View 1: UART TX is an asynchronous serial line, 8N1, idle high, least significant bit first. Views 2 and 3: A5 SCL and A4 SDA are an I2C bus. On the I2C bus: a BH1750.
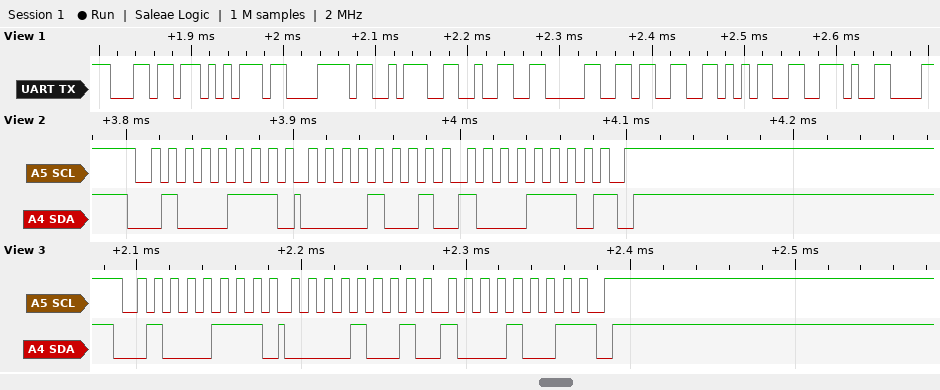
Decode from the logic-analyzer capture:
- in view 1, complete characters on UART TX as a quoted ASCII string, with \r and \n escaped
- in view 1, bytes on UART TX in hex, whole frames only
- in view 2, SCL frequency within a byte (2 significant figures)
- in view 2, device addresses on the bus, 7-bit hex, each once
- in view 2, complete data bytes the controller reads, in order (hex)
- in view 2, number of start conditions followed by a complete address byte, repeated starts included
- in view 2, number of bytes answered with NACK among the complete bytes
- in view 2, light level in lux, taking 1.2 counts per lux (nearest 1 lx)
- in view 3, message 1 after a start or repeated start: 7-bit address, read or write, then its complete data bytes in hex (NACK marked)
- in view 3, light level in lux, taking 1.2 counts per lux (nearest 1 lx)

"lux:2035."
6C 75 78 3A 32 30 33 35 2E
100 kHz
0x23
09 8E
1
1
2038 lx
0x23 read: 09 89 NACK
2034 lx
